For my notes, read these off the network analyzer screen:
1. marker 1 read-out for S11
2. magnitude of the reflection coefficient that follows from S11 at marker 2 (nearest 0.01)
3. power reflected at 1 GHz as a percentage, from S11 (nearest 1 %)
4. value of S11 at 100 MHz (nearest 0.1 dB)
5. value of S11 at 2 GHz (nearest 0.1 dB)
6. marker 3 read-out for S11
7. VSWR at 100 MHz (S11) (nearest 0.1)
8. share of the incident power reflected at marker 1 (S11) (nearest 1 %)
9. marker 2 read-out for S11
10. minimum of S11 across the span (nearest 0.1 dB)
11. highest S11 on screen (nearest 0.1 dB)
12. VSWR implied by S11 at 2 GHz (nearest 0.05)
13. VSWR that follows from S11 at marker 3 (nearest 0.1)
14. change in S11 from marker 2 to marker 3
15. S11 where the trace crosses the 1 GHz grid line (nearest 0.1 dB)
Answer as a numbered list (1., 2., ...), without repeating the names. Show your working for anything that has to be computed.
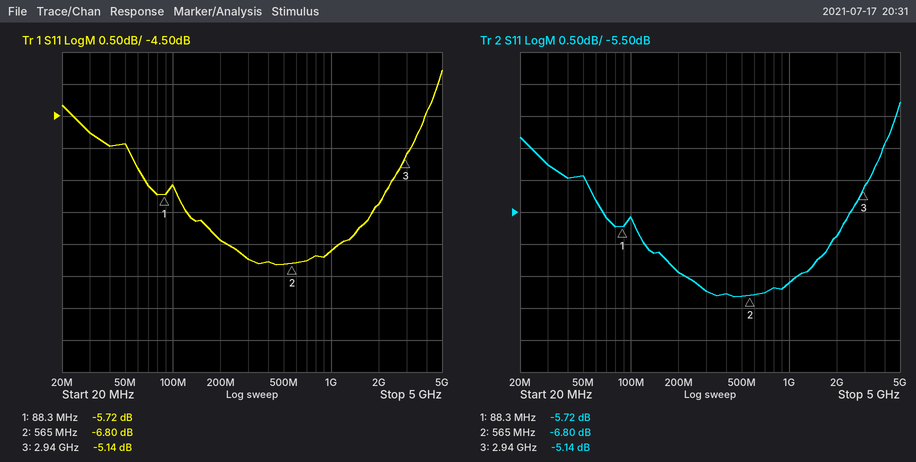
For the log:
1. -5.72 dB
2. 10^(-6.8/20) ≈ 0.46
3. 10^(-6.6/10) ≈ 22 %
4. -5.6 dB
5. -5.9 dB
6. -5.14 dB
7. |Γ| = 10^(-5.6/20) = 0.5248; VSWR = (1 + 0.5248)/(1 − 0.5248) ≈ 3.2
8. 10^(-5.72/10) ≈ 27 %
9. -6.80 dB
10. -6.8 dB
11. -3.8 dB
12. |Γ| = 10^(-5.9/20) = 0.5070; VSWR = (1 + 0.5070)/(1 − 0.5070) ≈ 3.06, so 3.05 to the nearest 0.05
13. (1 + 0.5534)/(1 − 0.5534) ≈ 3.5
14. -5.14 − (-6.8) = 1.66 dB
15. -6.6 dB
